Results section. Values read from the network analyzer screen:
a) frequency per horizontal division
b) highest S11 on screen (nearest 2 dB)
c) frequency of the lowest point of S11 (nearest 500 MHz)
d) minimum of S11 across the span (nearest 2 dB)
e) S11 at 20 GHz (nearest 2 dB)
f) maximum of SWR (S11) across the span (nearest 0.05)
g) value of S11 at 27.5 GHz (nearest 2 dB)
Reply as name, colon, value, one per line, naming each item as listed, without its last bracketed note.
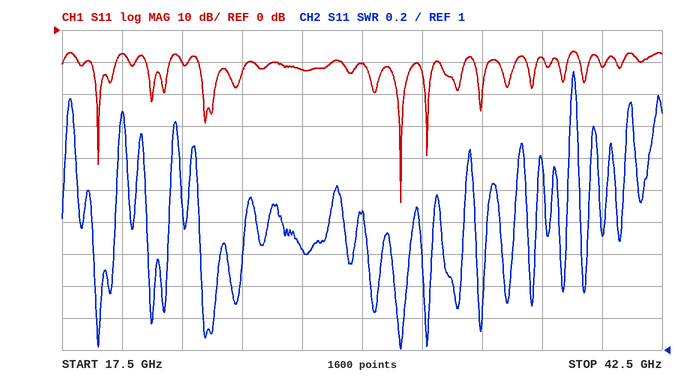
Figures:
frequency per horizontal division: 2.5 GHz
highest S11 on screen: -6 dB
frequency of the lowest point of S11: 31.5 GHz
minimum of S11 across the span: -54 dB
S11 at 20 GHz: -8 dB
maximum of SWR (S11) across the span: 2.75
value of S11 at 27.5 GHz: -12 dB
